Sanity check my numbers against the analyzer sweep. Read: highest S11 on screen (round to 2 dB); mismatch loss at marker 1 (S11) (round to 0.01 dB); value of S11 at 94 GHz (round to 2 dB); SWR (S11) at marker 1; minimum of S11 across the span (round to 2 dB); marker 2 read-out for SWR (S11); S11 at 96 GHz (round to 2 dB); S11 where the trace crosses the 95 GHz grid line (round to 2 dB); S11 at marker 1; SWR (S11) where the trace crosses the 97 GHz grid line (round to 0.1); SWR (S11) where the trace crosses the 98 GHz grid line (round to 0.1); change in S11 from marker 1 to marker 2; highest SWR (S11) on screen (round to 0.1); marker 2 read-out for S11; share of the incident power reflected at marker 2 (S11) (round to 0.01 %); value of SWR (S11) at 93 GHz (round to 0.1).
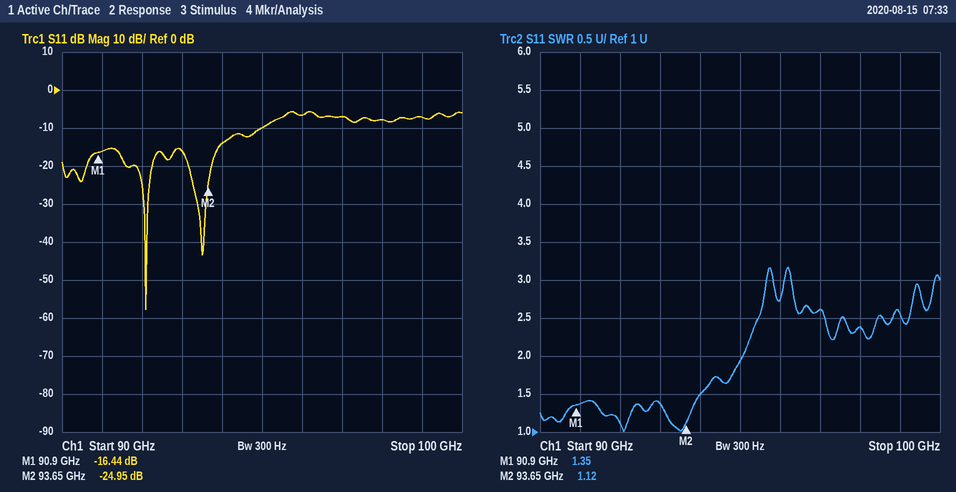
-6 dB
0.10 dB
-14 dB
1.35
-58 dB
1.12
-6 dB
-10 dB
-16.44 dB
2.6
2.4
-8.51 dB
3.2
-24.95 dB
0.32 %
1.4
